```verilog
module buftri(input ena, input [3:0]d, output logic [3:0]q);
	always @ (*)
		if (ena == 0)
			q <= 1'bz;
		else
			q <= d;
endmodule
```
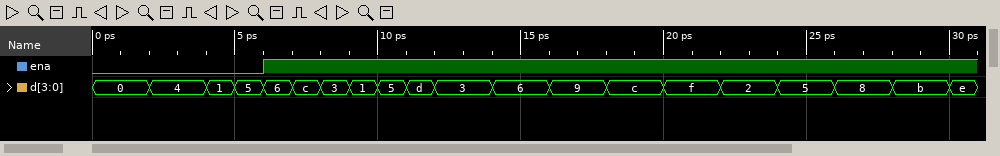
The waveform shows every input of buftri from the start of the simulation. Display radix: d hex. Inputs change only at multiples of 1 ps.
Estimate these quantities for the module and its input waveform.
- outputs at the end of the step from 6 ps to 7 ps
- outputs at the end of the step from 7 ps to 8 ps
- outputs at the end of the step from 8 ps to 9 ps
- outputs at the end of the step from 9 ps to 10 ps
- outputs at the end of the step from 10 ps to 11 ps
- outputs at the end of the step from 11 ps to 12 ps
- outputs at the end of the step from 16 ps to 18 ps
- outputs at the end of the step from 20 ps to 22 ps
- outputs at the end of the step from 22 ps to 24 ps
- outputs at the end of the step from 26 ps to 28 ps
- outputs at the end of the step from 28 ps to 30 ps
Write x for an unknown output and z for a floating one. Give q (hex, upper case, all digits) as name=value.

q=6
q=C
q=3
q=1
q=5
q=D
q=9
q=F
q=2
q=8
q=B
